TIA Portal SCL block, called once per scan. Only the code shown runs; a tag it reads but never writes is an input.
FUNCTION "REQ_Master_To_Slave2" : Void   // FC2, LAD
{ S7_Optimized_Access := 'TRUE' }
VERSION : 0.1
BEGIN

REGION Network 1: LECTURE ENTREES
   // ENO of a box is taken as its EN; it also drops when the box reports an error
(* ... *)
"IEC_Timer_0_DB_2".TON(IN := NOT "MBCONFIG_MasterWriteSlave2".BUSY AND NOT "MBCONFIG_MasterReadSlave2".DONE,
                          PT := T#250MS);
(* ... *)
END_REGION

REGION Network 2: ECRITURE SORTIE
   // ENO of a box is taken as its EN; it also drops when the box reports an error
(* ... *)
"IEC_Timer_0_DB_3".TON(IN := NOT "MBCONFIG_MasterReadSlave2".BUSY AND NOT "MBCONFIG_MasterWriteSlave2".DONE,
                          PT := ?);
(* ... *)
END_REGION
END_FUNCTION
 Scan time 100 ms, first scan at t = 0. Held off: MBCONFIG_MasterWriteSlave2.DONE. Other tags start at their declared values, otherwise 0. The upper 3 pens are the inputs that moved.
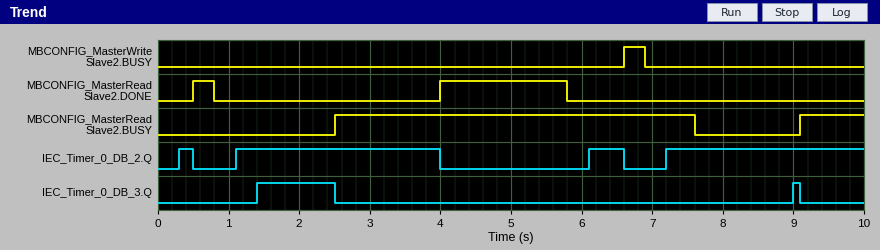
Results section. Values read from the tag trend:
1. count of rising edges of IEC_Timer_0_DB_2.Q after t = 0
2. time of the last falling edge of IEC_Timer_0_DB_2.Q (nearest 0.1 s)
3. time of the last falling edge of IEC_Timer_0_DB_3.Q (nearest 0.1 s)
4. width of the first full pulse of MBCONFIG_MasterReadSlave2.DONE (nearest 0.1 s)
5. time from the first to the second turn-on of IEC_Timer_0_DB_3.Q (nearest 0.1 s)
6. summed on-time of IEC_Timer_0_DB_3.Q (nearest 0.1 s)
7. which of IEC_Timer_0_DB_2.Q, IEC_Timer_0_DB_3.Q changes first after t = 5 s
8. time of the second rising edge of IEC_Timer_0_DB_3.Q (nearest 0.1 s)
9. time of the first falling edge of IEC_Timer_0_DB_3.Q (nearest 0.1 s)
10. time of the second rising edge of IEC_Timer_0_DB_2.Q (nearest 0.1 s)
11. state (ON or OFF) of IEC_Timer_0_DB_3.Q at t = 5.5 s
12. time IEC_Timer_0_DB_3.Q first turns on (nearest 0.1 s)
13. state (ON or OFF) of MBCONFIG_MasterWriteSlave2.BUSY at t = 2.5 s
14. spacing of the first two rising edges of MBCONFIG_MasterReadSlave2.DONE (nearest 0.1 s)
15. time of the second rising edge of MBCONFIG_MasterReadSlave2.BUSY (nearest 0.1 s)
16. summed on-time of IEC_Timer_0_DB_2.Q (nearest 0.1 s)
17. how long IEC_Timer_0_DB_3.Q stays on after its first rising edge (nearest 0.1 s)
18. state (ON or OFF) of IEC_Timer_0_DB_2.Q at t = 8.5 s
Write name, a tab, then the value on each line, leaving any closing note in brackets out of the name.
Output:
count of rising edges of IEC_Timer_0_DB_2.Q after t = 0	4
time of the last falling edge of IEC_Timer_0_DB_2.Q	6.6 s
time of the last falling edge of IEC_Timer_0_DB_3.Q	9.1 s
width of the first full pulse of MBCONFIG_MasterReadSlave2.DONE	0.3 s
time from the first to the second turn-on of IEC_Timer_0_DB_3.Q	7.6 s
summed on-time of IEC_Timer_0_DB_3.Q	1.2 s
which of IEC_Timer_0_DB_2.Q, IEC_Timer_0_DB_3.Q changes first after t = 5 s	IEC_Timer_0_DB_2.Q
time of the second rising edge of IEC_Timer_0_DB_3.Q	9.0 s
time of the first falling edge of IEC_Timer_0_DB_3.Q	2.5 s
time of the second rising edge of IEC_Timer_0_DB_2.Q	1.1 s
state (ON or OFF) of IEC_Timer_0_DB_3.Q at t = 5.5 s	OFF
time IEC_Timer_0_DB_3.Q first turns on	1.4 s
state (ON or OFF) of MBCONFIG_MasterWriteSlave2.BUSY at t = 2.5 s	OFF
spacing of the first two rising edges of MBCONFIG_MasterReadSlave2.DONE	3.5 s
time of the second rising edge of MBCONFIG_MasterReadSlave2.BUSY	9.1 s
summed on-time of IEC_Timer_0_DB_2.Q	6.4 s
how long IEC_Timer_0_DB_3.Q stays on after its first rising edge	1.1 s
state (ON or OFF) of IEC_Timer_0_DB_2.Q at t = 8.5 s	ON
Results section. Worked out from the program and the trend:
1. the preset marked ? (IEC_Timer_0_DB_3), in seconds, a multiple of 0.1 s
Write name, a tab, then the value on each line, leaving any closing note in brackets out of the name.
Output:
the preset marked ? (IEC_Timer_0_DB_3), in seconds, a multiple of 0.1 s	1.4 s
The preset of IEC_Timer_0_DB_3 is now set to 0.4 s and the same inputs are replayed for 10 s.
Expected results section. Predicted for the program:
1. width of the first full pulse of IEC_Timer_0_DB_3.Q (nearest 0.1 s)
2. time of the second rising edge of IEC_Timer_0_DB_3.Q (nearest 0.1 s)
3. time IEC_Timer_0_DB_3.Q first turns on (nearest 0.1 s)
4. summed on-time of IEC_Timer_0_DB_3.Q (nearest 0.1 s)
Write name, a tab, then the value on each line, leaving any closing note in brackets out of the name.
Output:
width of the first full pulse of IEC_Timer_0_DB_3.Q	2.1 s
time of the second rising edge of IEC_Timer_0_DB_3.Q	8.0 s
time IEC_Timer_0_DB_3.Q first turns on	0.4 s
summed on-time of IEC_Timer_0_DB_3.Q	3.2 s
